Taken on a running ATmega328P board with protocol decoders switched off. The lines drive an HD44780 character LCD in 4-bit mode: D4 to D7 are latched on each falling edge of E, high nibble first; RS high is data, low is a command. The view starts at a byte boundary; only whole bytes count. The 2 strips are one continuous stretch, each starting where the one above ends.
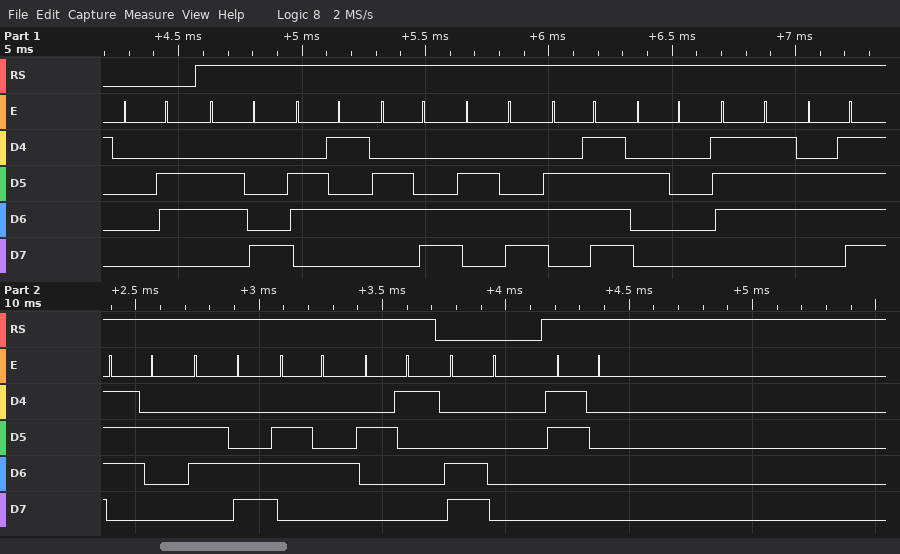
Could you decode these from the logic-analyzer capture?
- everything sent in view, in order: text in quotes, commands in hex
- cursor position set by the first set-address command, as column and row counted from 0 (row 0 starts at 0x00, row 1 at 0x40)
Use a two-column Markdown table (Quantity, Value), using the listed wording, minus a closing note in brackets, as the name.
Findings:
| Quantity | Value |
|---|---|
| everything sent in view, in order: text in quotes, commands in hex | 0x06 "hello world!" 0xC0 "0" |
| cursor position set by the first set-address command, as column and row counted from 0 | column 0, row 1 |
